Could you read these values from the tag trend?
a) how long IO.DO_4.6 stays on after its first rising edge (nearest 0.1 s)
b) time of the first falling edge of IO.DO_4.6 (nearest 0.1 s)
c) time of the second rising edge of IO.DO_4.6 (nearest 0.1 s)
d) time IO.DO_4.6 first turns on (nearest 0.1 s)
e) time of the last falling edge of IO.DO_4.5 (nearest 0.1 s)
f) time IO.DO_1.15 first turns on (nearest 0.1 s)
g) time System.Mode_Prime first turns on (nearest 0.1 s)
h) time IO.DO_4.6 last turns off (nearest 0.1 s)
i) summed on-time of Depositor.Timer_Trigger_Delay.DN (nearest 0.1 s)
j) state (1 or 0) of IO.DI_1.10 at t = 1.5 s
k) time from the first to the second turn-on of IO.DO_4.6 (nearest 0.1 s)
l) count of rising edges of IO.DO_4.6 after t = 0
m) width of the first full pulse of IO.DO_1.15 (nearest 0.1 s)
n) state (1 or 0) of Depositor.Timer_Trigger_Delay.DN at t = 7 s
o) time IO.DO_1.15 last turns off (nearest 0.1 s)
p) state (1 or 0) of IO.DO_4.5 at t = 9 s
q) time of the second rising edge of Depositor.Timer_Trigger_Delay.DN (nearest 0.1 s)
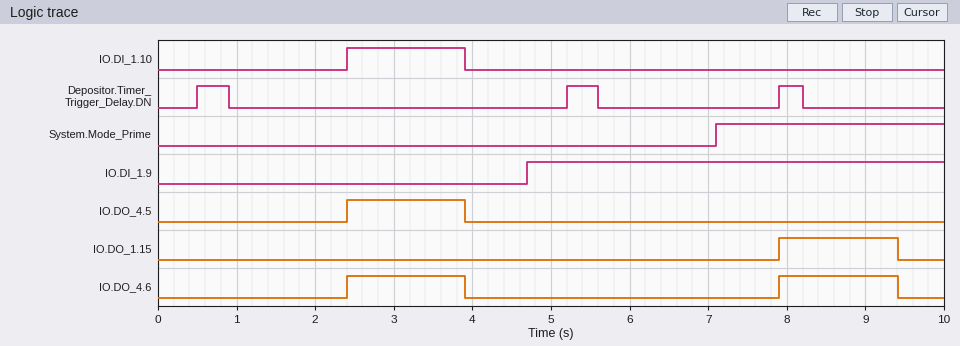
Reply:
1.5 s
3.9 s
7.9 s
2.4 s
3.9 s
7.9 s
7.1 s
9.4 s
1.1 s
0
5.5 s
2
1.5 s
0
9.4 s
0
5.2 s
